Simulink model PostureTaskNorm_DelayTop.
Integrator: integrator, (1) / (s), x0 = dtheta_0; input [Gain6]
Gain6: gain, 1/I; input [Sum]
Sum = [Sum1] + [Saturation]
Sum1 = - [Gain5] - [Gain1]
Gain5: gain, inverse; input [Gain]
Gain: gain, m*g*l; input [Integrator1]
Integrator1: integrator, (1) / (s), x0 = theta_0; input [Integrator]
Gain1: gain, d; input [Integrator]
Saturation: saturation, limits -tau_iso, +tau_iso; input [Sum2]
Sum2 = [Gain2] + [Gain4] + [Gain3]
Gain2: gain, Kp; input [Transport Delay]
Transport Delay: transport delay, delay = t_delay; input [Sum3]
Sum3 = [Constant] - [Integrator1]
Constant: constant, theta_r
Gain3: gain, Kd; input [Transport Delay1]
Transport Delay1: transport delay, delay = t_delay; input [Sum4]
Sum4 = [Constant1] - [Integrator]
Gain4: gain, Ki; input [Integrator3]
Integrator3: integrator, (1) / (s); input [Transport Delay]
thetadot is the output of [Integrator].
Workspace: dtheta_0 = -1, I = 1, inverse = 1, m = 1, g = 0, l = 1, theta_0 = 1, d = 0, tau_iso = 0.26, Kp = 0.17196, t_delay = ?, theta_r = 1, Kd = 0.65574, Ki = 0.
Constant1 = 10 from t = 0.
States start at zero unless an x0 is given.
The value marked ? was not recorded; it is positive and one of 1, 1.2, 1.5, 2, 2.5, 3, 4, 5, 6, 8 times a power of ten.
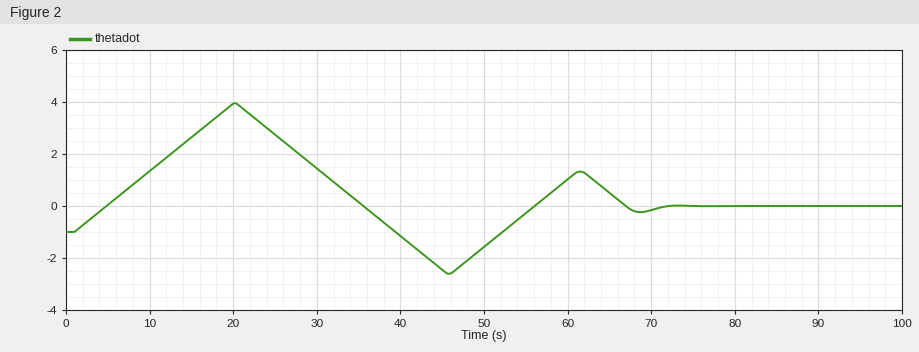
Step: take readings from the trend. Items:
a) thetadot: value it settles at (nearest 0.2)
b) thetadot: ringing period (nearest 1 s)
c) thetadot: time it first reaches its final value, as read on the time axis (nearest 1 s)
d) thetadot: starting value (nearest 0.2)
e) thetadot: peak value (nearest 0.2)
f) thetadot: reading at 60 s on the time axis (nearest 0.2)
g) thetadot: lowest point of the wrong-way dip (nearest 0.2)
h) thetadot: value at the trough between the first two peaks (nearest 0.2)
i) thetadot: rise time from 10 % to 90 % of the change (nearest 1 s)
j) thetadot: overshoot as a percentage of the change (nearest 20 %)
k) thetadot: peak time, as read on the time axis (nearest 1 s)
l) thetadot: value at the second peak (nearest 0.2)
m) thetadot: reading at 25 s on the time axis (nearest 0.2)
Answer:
0.0
41 s
5 s
-1.0
4.0
1.0
-2.6
-2.6
3 s
400 %
20 s
1.4
2.8
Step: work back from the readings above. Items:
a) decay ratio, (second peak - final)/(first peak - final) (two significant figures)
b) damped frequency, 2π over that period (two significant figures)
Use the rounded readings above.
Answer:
0.35
0.15 rad/s
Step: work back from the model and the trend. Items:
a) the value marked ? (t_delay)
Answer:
1
